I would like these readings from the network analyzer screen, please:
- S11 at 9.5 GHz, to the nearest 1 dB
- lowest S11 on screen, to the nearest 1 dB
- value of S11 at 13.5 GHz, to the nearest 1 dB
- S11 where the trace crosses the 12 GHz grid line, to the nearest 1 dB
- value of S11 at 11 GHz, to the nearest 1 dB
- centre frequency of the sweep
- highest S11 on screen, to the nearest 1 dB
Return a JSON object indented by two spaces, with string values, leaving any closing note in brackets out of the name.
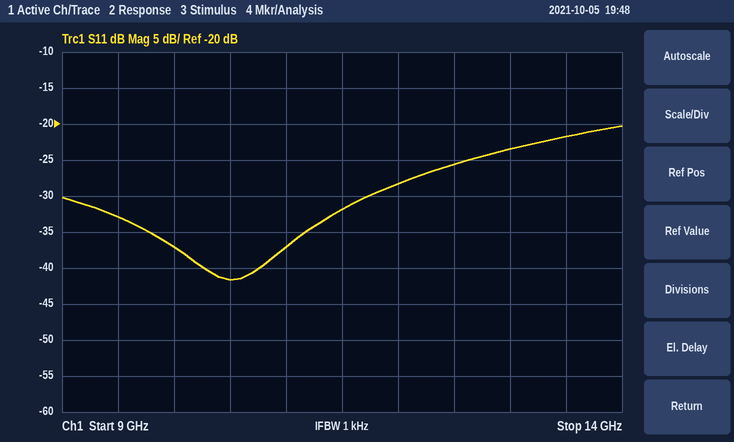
{
  "S11 at 9.5 GHz, to the nearest 1 dB": "-33 dB",
  "lowest S11 on screen, to the nearest 1 dB": "-42 dB",
  "value of S11 at 13.5 GHz, to the nearest 1 dB": "-22 dB",
  "S11 where the trace crosses the 12 GHz grid line, to the nearest 1 dB": "-28 dB",
  "value of S11 at 11 GHz, to the nearest 1 dB": "-37 dB",
  "centre frequency of the sweep": "11.5 GHz",
  "highest S11 on screen, to the nearest 1 dB": "-20 dB"
}
